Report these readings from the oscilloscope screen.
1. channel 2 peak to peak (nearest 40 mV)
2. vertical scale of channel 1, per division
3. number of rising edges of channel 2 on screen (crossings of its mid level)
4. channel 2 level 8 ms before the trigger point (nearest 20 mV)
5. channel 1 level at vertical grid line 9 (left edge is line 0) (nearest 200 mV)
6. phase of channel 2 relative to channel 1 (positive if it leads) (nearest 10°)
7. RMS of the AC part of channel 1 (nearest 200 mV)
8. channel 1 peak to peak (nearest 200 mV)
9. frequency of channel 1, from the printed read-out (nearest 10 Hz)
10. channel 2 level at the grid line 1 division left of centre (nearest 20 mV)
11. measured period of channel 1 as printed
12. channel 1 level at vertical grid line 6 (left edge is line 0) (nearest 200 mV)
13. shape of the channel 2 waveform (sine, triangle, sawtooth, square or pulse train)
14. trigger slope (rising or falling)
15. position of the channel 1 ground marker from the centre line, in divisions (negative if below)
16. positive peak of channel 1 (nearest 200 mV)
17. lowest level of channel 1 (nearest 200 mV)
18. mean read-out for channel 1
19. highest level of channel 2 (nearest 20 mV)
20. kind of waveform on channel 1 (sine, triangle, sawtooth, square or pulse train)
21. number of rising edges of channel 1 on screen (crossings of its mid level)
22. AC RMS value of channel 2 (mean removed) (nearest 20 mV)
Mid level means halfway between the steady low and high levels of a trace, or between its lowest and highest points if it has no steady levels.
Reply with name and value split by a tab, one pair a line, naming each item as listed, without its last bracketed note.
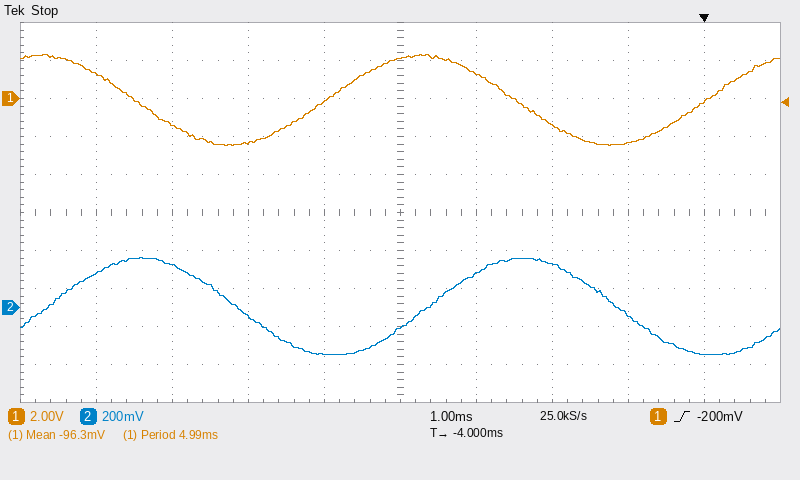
channel 2 peak to peak	520 mV
vertical scale of channel 1, per division	2 V
number of rising edges of channel 2 on screen	2
channel 2 level 8 ms before the trigger point	180 mV
channel 1 level at vertical grid line 9 (left edge is line 0)	-200 mV
phase of channel 2 relative to channel 1 (positive if it leads)	-100°
RMS of the AC part of channel 1	1.6 V
channel 1 peak to peak	4.8 V
frequency of channel 1, from the printed read-out	200 Hz
channel 2 level at the grid line 1 division left of centre	-240 mV
measured period of channel 1 as printed	4.99 ms
channel 1 level at vertical grid line 6 (left edge is line 0)	1.4 V
shape of the channel 2 waveform	sine
trigger slope	rising
position of the channel 1 ground marker from the centre line, in divisions	+3.0 div
positive peak of channel 1	2.4 V
lowest level of channel 1	-2.4 V
mean read-out for channel 1	-96.3 mV
highest level of channel 2	260 mV
kind of waveform on channel 1	sine
number of rising edges of channel 1 on screen	2
AC RMS value of channel 2 (mean removed)	180 mV
